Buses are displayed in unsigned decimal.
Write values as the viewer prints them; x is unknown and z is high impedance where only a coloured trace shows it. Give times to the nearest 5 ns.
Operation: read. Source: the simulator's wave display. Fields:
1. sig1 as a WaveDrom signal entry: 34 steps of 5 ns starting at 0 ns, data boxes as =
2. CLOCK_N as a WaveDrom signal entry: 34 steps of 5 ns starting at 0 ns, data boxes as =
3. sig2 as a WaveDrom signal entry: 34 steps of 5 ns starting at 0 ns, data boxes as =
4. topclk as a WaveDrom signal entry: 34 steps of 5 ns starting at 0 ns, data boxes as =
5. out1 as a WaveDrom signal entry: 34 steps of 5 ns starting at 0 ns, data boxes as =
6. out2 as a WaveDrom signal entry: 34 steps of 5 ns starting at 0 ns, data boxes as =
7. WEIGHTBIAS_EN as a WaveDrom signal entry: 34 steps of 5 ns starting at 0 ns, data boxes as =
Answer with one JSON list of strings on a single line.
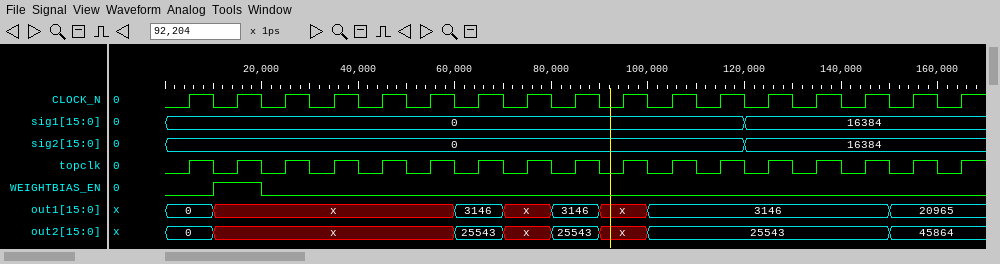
["{name: 'sig1', wave: '=.......................=.........', data: '0 16384'}", "{name: 'CLOCK_N', wave: '0101010101010101010101010101010101'}", "{name: 'sig2', wave: '=.......................=.........', data: '0 16384'}", "{name: 'topclk', wave: '0101010101010101010101010101010101'}", "{name: 'out1', wave: '=.x.........=.x.=.x.=.........=...', data: '0 3146 3146 3146 20965'}", "{name: 'out2', wave: '=.x.........=.x.=.x.=.........=...', data: '0 25543 25543 25543 45864'}", "{name: 'WEIGHTBIAS_EN', wave: '0.1.0.............................'}"]
